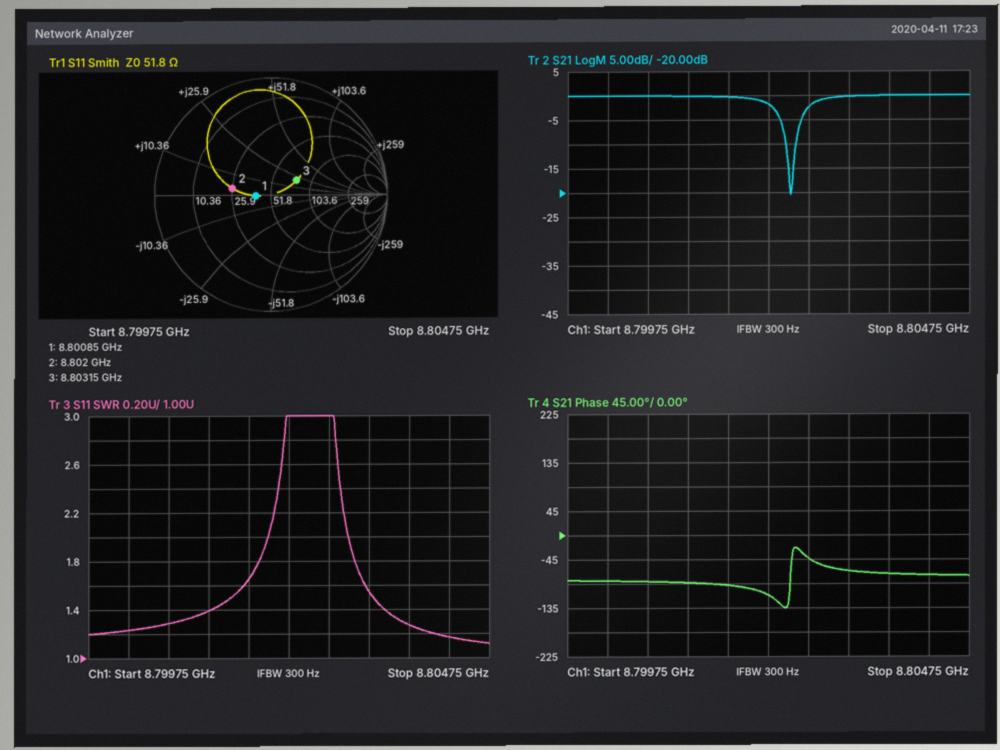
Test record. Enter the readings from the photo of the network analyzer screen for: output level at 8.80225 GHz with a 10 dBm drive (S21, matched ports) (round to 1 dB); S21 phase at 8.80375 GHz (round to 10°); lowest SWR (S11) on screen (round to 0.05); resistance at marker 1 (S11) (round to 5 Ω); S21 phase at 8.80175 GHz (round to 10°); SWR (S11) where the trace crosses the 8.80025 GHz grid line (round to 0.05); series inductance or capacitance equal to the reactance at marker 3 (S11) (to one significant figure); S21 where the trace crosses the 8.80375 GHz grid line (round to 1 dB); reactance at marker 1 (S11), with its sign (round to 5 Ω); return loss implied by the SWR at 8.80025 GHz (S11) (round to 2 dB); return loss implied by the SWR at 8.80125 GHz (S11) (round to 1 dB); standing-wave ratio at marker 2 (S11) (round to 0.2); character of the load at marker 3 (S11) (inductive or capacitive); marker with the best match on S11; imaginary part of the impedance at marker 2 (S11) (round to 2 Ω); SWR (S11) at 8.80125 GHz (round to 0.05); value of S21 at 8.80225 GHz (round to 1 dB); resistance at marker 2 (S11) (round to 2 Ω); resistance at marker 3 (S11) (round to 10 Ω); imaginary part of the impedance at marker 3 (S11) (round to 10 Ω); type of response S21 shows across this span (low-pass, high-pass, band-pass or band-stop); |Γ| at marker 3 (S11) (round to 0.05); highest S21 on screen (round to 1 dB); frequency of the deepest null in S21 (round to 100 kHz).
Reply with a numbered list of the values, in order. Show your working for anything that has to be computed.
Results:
1. 10 dBm + (-2 dB) = 8 dBm
2. -70°
3. 1.10
4. 40 Ω
5. -90°
6. 1.25
7. L = 20 Ω/(2π × 8.80315 GHz) ≈ 362 pH, so 400 pH to one significant figure
8. 0 dB
9. 0 Ω
10. −20 log10((1.25 − 1)/(1.25 + 1)) ≈ 19.1 dB, so 20 dB to the nearest 2 dB
11. −20 log10((1.4 − 1)/(1.4 + 1)) ≈ 16 dB
12. 2.0
13. inductive
14. marker 1
15. +4 Ω
16. 1.40
17. -2 dB
18. 26 Ω
19. 80 Ω
20. +20 Ω
21. band-stop
22. 0.25
23. 0 dB
24. 8.8025 GHz
